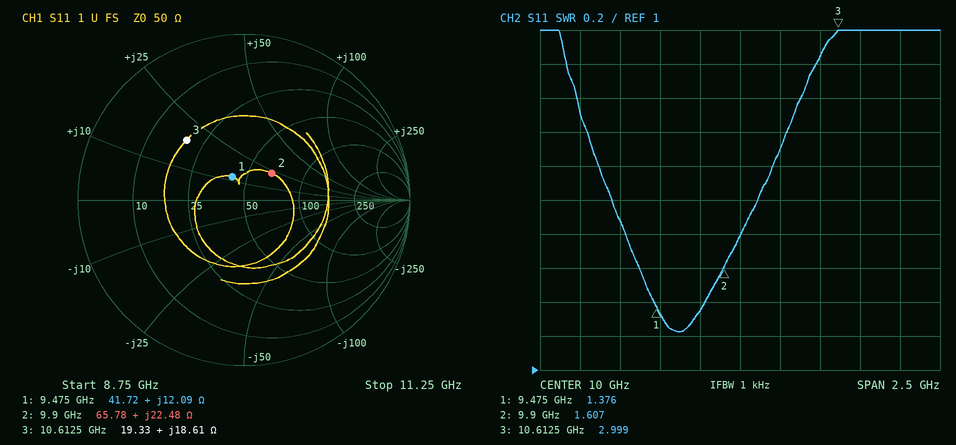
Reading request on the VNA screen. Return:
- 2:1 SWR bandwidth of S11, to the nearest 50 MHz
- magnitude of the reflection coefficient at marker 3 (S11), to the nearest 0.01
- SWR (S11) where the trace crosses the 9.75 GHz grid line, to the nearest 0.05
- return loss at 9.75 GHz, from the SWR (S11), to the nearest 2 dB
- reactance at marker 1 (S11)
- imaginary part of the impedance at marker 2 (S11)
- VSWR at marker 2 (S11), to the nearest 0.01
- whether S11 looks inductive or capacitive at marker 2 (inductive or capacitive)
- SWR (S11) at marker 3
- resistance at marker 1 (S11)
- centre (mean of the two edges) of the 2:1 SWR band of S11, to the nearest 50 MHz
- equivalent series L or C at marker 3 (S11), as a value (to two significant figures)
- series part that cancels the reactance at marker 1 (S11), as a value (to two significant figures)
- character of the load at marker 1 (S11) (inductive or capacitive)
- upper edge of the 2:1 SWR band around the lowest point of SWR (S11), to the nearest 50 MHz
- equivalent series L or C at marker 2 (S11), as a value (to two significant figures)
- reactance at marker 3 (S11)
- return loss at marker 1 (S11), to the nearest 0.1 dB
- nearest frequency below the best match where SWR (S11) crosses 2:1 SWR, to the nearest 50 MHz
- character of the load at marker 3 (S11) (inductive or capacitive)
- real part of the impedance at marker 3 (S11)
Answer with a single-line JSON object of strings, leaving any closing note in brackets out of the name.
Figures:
{"2:1 SWR bandwidth of S11, to the nearest 50 MHz": "900 MHz", "magnitude of the reflection coefficient at marker 3 (S11), to the nearest 0.01": "0.50", "SWR (S11) where the trace crosses the 9.75 GHz grid line, to the nearest 0.05": "1.35", "return loss at 9.75 GHz, from the SWR (S11), to the nearest 2 dB": "16 dB", "reactance at marker 1": "+12.09 Ω", "imaginary part of the impedance at marker 2": "+22.48 Ω", "VSWR at marker 2 (S11), to the nearest 0.01": "1.61", "whether S11 looks inductive or capacitive at marker 2": "inductive", "SWR (S11) at marker 3": "2.999", "resistance at marker 1": "41.72 Ω", "centre (mean of the two edges) of the 2:1 SWR band of S11, to the nearest 50 MHz": "9.65 GHz", "equivalent series L or C at marker 3 (S11), as a value": "280 pH", "series part that cancels the reactance at marker 1 (S11), as a value": "1.4 pF", "character of the load at marker 1 (S11)": "inductive", "upper edge of the 2:1 SWR band around the lowest point of SWR (S11), to the nearest 50 MHz": "10.10 GHz", "equivalent series L or C at marker 2 (S11), as a value": "360 pH", "reactance at marker 3": "+18.61 Ω", "return loss at marker 1 (S11), to the nearest 0.1 dB": "16.0 dB", "nearest frequency below the best match where SWR (S11) crosses 2:1 SWR, to the nearest 50 MHz": "9.20 GHz", "character of the load at marker 3 (S11)": "inductive", "real part of the impedance at marker 3": "19.33 Ω"}
